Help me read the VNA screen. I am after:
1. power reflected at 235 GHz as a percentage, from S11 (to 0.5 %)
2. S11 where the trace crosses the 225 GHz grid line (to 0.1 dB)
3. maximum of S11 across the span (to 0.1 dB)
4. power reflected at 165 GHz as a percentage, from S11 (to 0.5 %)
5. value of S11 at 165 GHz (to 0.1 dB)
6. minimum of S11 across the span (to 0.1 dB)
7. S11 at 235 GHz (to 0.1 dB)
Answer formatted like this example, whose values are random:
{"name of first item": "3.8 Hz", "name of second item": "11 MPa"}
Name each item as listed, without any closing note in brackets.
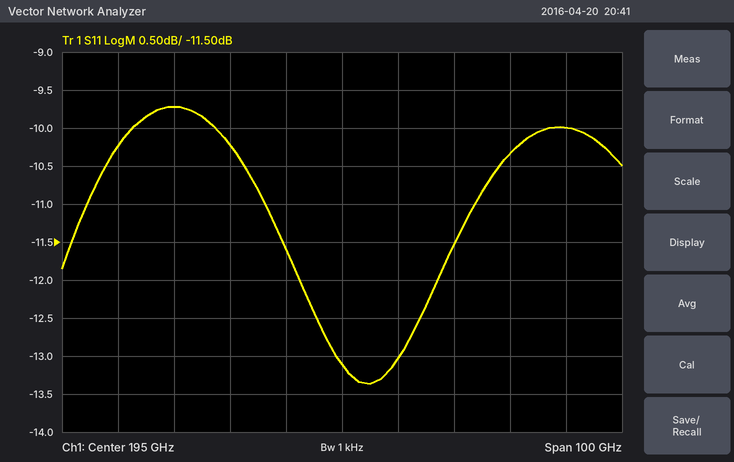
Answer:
{"power reflected at 235 GHz as a percentage, from S11": "10.0 %", "S11 where the trace crosses the 225 GHz grid line": "-10.3 dB", "maximum of S11 across the span": "-9.7 dB", "power reflected at 165 GHz as a percentage, from S11": "10.5 %", "value of S11 at 165 GHz": "-9.7 dB", "minimum of S11 across the span": "-13.4 dB", "S11 at 235 GHz": "-10.0 dB"}
